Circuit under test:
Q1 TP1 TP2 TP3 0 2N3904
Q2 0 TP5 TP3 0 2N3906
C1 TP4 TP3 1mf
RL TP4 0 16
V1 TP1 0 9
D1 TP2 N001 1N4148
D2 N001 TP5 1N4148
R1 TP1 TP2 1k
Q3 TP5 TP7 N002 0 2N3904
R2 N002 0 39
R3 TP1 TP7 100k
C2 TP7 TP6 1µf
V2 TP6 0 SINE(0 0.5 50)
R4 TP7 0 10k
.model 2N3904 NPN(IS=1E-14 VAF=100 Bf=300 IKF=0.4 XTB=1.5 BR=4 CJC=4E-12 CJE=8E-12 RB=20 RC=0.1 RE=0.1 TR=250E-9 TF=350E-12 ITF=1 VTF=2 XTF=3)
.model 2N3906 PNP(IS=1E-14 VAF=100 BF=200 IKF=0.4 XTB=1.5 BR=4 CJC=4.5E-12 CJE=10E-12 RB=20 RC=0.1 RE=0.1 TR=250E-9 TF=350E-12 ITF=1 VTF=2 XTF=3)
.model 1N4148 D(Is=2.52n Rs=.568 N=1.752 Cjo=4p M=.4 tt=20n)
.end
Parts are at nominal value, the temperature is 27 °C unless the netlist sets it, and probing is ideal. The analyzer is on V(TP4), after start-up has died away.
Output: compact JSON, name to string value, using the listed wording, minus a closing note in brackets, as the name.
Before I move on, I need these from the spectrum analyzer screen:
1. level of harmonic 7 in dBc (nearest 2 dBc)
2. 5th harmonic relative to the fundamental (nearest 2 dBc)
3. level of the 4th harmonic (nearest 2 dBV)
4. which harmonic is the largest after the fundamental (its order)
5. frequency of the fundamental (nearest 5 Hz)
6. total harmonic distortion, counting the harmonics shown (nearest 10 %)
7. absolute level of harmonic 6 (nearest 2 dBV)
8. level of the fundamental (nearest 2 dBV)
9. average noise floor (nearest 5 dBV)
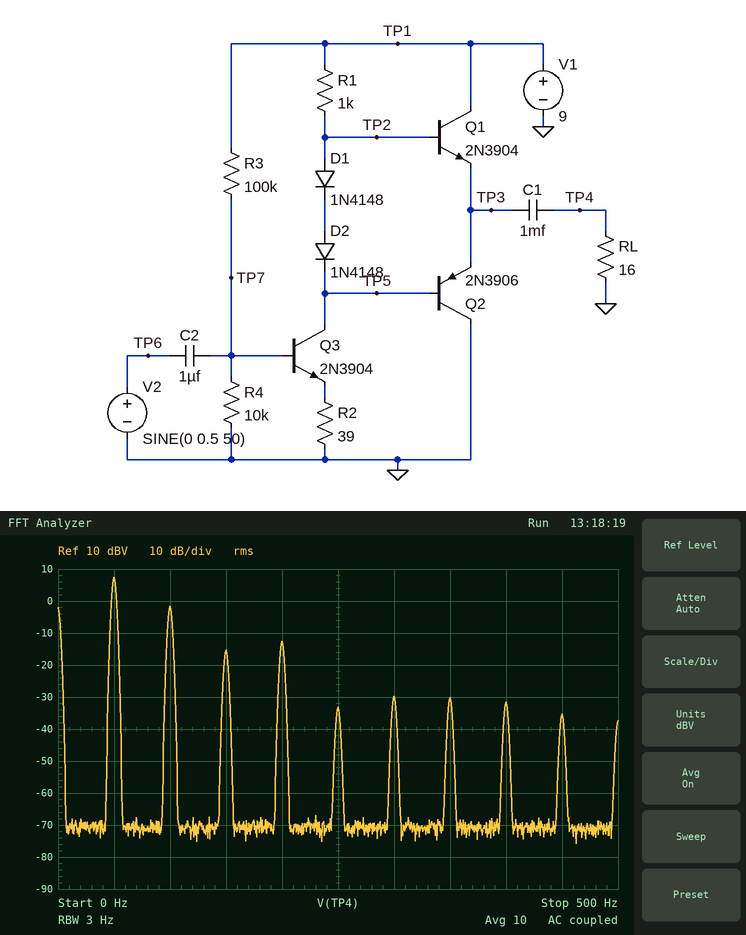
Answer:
{"level of harmonic 7 in dBc": "-38 dBc", "5th harmonic relative to the fundamental": "-40 dBc", "level of the 4th harmonic": "-12 dBV", "which harmonic is the largest after the fundamental": "2", "frequency of the fundamental": "50 Hz", "total harmonic distortion, counting the harmonics shown": "40 %", "absolute level of harmonic 6": "-30 dBV", "level of the fundamental": "8 dBV", "average noise floor": "-70 dBV"}
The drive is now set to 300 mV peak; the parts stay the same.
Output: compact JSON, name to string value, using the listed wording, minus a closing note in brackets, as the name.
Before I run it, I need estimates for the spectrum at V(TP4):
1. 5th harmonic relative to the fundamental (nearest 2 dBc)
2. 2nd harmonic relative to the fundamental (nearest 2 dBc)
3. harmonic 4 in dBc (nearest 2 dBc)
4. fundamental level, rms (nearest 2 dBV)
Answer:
{"5th harmonic relative to the fundamental": "-36 dBc", "2nd harmonic relative to the fundamental": "-12 dBc", "harmonic 4 in dBc": "-36 dBc", "fundamental level, rms": "6 dBV"}
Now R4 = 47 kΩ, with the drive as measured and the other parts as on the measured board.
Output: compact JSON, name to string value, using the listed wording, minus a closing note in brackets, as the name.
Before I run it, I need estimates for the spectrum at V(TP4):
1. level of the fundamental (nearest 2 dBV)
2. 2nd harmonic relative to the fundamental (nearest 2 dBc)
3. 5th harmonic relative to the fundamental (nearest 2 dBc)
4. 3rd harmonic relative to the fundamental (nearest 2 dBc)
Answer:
{"level of the fundamental": "8 dBV", "2nd harmonic relative to the fundamental": "-14 dBc", "5th harmonic relative to the fundamental": "-28 dBc", "3rd harmonic relative to the fundamental": "-16 dBc"}
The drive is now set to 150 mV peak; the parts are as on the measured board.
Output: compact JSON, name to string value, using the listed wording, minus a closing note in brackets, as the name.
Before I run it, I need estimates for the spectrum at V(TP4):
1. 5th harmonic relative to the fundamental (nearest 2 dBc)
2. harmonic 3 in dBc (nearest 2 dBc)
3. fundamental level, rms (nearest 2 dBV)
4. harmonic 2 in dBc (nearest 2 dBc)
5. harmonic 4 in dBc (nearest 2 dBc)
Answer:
{"5th harmonic relative to the fundamental": "-42 dBc", "harmonic 3 in dBc": "-34 dBc", "fundamental level, rms": "2 dBV", "harmonic 2 in dBc": "-22 dBc", "harmonic 4 in dBc": "-42 dBc"}
